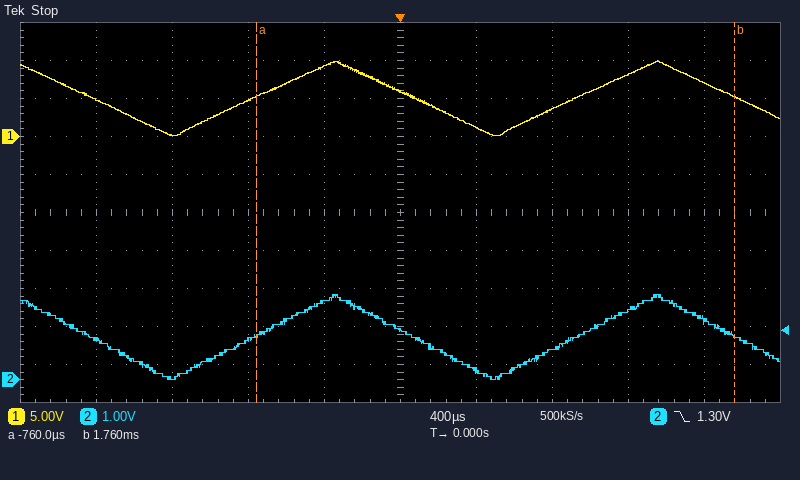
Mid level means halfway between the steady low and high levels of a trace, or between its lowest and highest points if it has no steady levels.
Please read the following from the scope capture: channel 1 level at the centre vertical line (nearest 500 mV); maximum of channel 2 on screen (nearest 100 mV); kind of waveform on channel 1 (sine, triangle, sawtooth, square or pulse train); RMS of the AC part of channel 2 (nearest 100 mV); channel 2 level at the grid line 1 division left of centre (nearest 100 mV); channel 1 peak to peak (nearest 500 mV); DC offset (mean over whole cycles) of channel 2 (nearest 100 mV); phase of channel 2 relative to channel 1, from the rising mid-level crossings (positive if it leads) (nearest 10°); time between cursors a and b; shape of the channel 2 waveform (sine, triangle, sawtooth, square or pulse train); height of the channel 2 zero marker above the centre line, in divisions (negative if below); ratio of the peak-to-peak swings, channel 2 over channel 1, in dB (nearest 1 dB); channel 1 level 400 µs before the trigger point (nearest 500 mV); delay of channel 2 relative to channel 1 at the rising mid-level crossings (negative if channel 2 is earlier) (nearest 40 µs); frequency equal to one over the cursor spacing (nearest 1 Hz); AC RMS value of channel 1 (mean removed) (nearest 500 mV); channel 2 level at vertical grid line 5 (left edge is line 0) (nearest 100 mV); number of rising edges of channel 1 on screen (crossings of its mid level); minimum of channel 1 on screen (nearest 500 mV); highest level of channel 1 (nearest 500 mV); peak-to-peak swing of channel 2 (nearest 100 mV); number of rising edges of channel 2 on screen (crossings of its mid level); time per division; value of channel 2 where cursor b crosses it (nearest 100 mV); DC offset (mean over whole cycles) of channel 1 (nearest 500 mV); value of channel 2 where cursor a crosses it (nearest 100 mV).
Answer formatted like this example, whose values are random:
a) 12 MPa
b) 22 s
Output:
a) 6.0 V
b) 2.2 V
c) triangle
d) 600 mV
e) 2.0 V
f) 10.0 V
g) 1.1 V
h) 0°
i) 2.52 ms
j) triangle
k) -4.4 div
l) -13 dB
m) 9.0 V
n) 0 µs
o) 397 Hz
p) 3.0 V
q) 1.3 V
r) 2
s) 0.0 V
t) 10.0 V
u) 2.2 V
v) 2
w) 400 µs
x) 1.2 V
y) 5.0 V
z) 1.2 V
